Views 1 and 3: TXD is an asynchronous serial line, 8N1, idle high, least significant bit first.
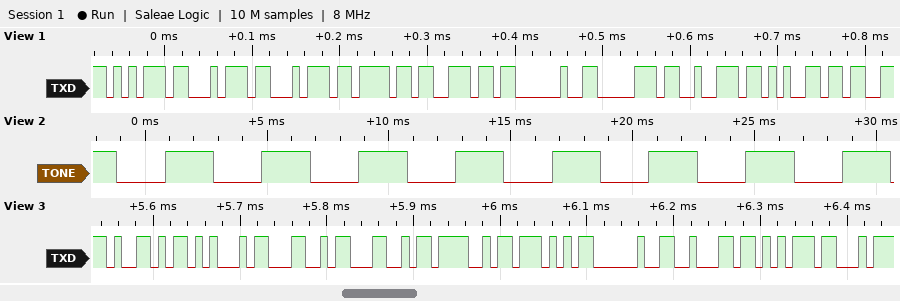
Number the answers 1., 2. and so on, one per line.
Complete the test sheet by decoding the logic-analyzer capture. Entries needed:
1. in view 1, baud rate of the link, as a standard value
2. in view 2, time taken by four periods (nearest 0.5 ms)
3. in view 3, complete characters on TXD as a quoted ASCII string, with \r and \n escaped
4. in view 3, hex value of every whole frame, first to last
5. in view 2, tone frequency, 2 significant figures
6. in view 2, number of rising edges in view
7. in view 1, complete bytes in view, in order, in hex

1. 115200 baud
2. 16.0 ms
3. "YELLOW bu"
4. 59 45 4C 4C 4F 57 20 62 75
5. 250 Hz
6. 8
7. 0x75 0x74 0x74 0x6F 0x6E 0x20 0x70 0x72 0x65
